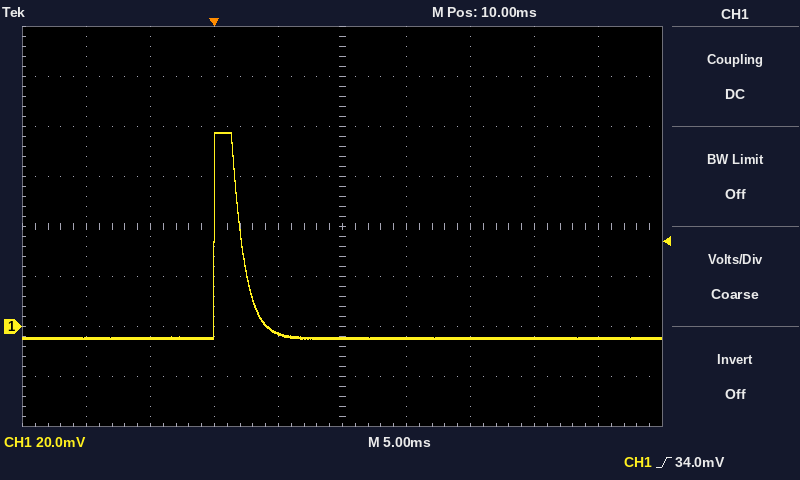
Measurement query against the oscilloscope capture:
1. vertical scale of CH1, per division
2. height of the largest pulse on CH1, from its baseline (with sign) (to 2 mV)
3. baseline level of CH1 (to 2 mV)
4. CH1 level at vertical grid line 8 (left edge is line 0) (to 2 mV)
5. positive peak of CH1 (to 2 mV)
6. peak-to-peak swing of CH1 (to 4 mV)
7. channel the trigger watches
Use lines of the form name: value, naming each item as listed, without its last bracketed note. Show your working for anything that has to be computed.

vertical scale of CH1, per division: 20 mV
height of the largest pulse on CH1, from its baseline (with sign): 78 mV − (-4 mV) = +82 mV
baseline level of CH1: -4 mV
CH1 level at vertical grid line 8 (left edge is line 0): -4 mV
positive peak of CH1: 78 mV
peak-to-peak swing of CH1: 84 mV
channel the trigger watches: CH1
